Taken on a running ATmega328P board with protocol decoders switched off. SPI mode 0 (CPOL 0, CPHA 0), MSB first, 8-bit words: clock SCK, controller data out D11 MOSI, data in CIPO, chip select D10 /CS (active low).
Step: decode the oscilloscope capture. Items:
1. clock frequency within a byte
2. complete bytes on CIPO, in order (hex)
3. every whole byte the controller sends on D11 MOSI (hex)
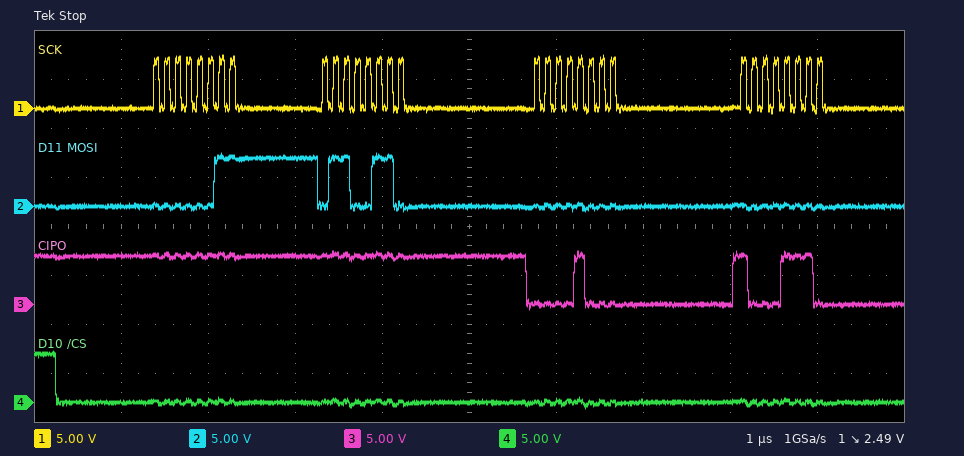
8 MHz
0xFF 0xFF 0x08 0x8E
0x03 0x66 0x00 0x00
